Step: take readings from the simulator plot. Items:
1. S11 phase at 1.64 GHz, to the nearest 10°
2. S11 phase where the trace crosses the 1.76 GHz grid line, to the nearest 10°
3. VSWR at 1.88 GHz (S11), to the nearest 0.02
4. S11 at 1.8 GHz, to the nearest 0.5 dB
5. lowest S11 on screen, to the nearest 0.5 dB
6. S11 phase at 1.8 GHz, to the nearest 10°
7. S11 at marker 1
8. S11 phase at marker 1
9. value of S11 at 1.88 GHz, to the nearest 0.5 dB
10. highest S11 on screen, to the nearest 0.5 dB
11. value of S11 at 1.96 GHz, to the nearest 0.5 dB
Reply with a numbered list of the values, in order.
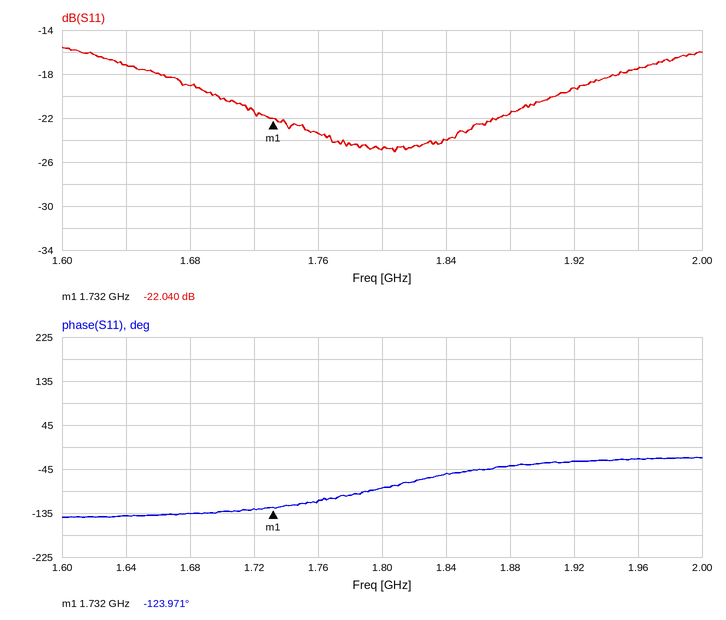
1. -140°
2. -110°
3. 1.18
4. -25.0 dB
5. -25.0 dB
6. -80°
7. -22.040 dB
8. -123.971°
9. -21.5 dB
10. -15.5 dB
11. -17.5 dB
